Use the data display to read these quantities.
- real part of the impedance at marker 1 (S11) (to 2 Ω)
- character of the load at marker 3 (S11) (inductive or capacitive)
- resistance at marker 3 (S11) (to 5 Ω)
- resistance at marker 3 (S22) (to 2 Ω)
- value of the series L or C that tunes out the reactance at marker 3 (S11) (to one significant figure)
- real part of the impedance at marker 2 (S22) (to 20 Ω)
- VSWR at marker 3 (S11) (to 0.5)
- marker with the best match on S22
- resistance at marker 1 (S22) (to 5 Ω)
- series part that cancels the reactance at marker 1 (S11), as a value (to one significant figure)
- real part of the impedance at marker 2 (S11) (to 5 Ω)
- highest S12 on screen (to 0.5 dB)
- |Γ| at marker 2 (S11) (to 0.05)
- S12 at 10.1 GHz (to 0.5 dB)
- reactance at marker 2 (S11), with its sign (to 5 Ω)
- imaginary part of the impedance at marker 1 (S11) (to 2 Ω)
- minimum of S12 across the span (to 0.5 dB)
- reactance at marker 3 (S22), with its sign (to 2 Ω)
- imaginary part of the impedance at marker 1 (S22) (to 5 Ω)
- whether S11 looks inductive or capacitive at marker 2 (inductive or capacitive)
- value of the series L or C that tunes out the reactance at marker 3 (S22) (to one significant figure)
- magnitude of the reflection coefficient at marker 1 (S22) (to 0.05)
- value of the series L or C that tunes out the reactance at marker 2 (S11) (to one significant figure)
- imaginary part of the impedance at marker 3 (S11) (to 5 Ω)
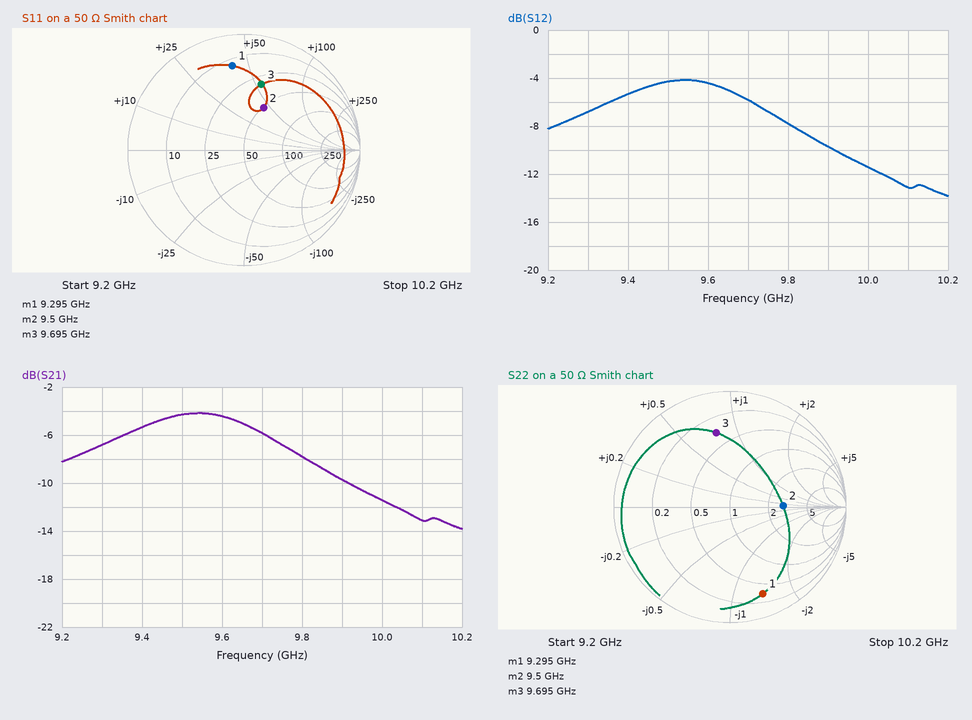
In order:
14 Ω
inductive
30 Ω
18 Ω
300 fF
140 Ω
4.0
marker 2
15 Ω
400 fF
50 Ω
-4.0 dB
0.40
-13.0 dB
+45 Ω
+42 Ω
-14.0 dB
+38 Ω
-70 Ω
inductive
400 fF
0.80
400 fF
+55 Ω
